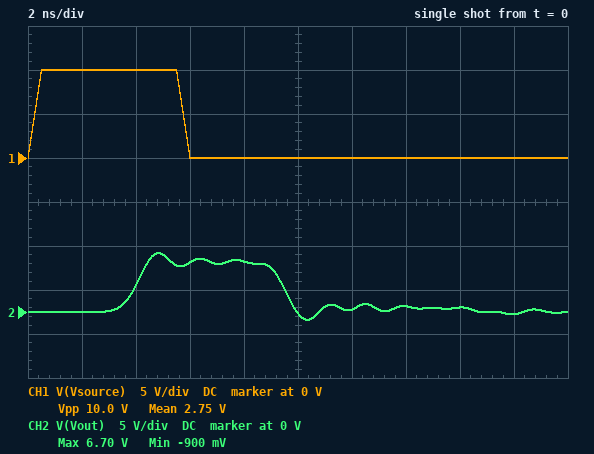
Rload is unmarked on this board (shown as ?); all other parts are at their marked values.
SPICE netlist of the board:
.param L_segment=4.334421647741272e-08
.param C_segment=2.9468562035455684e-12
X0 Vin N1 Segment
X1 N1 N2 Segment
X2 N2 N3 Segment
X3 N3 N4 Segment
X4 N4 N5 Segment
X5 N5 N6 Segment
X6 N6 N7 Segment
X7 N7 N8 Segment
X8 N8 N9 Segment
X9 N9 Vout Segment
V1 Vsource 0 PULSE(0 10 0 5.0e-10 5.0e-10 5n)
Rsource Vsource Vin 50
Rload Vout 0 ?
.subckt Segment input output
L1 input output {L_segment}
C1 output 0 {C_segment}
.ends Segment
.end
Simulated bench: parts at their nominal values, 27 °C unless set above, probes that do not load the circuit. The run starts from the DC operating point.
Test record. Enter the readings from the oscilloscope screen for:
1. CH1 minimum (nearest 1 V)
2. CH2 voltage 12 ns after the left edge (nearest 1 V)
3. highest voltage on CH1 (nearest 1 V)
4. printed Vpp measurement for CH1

0 V
0 V
10 V
10.0 V
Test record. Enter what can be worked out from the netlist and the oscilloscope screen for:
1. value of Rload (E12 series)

82 Ω
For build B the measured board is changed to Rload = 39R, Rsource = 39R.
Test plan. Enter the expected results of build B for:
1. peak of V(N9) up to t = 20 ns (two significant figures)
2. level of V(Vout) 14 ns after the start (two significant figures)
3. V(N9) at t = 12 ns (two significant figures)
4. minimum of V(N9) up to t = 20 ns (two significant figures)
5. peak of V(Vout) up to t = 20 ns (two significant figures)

7.1 V
1.1 V
2.6 V
-3.0 V
4.3 V
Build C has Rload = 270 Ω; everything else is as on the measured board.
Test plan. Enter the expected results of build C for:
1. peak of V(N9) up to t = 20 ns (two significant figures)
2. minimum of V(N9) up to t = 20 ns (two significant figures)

11 V
-2.8 V
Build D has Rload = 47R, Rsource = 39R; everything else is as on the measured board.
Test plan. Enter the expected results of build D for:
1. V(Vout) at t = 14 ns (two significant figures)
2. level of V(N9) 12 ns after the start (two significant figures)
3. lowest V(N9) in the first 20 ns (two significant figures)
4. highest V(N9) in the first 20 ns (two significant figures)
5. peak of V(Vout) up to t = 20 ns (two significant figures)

1.1 V
2.5 V
-2.7 V
7.3 V
4.9 V
